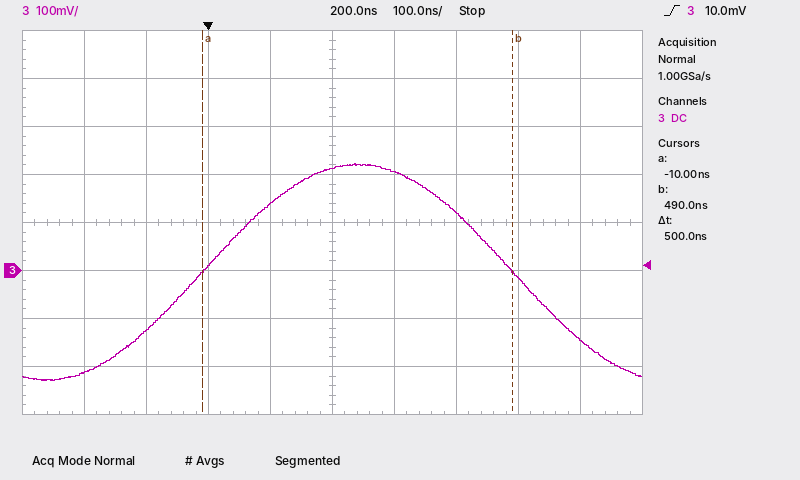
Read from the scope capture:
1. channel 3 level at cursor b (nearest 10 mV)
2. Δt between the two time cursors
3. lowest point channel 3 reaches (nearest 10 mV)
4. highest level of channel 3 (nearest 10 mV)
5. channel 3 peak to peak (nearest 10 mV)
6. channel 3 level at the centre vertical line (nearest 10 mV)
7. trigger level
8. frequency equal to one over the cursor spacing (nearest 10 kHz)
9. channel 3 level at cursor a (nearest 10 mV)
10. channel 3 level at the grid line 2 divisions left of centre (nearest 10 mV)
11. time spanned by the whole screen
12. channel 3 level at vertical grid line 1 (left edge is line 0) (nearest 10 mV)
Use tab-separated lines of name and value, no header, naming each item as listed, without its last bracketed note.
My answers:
channel 3 level at cursor b	0 mV
Δt between the two time cursors	500 ns
lowest point channel 3 reaches	-230 mV
highest level of channel 3	220 mV
channel 3 peak to peak	450 mV
channel 3 level at the centre vertical line	210 mV
trigger level	10.0 mV
frequency equal to one over the cursor spacing	2.00 MHz
channel 3 level at cursor a	0 mV
channel 3 level at the grid line 2 divisions left of centre	10 mV
time spanned by the whole screen	1 µs
channel 3 level at vertical grid line 1 (left edge is line 0)	-210 mV
